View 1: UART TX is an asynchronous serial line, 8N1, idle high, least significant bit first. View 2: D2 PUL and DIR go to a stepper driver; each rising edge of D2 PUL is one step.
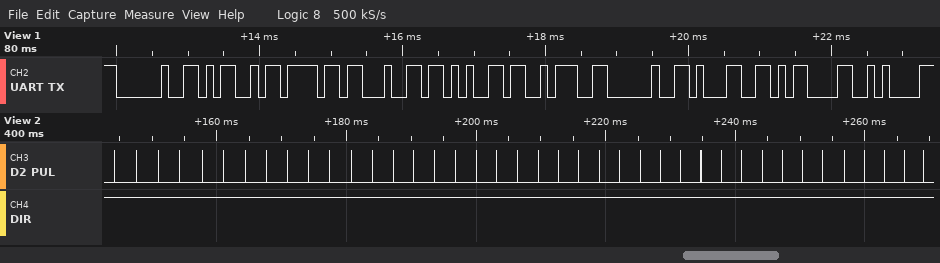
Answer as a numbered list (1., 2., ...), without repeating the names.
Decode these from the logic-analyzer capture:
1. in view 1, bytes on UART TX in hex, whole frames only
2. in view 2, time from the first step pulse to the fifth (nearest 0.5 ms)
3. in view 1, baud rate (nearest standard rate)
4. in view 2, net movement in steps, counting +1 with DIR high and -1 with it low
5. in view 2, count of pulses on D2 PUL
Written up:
1. 20 4D 6F 64 65 3A 20 31 0D 0A
2. 13.5 ms
3. 9600 baud
4. +40
5. 40
